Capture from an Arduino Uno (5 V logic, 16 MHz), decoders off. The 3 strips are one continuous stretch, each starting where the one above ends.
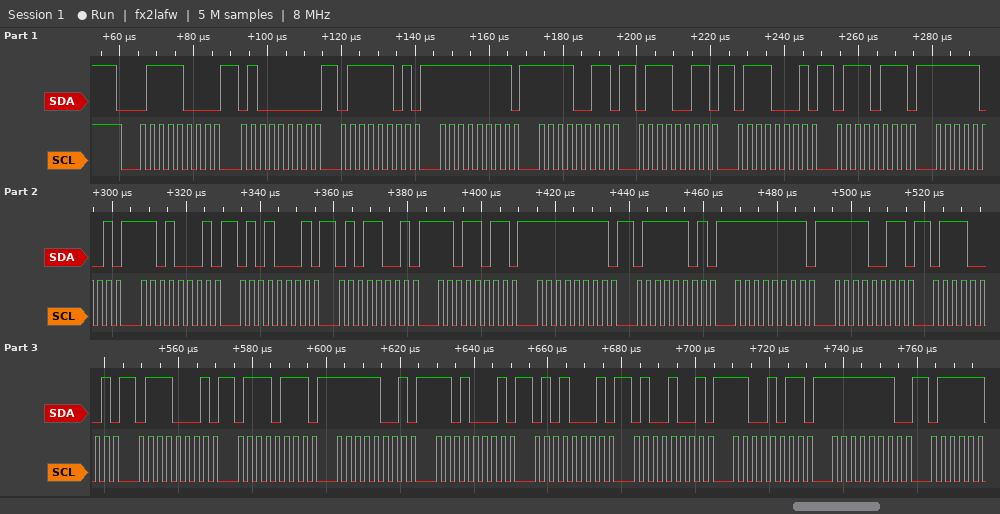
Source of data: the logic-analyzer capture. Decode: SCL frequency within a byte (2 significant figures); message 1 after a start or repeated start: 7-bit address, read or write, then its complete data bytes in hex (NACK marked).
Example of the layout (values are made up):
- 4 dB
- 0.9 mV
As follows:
- 400 kHz
- 0x3C write: 40 7D FF F3 73 71 77 F9 D1 51 59 DB FF 7D FF F3 71 71 77 F9 D1 51 49 CB FE
